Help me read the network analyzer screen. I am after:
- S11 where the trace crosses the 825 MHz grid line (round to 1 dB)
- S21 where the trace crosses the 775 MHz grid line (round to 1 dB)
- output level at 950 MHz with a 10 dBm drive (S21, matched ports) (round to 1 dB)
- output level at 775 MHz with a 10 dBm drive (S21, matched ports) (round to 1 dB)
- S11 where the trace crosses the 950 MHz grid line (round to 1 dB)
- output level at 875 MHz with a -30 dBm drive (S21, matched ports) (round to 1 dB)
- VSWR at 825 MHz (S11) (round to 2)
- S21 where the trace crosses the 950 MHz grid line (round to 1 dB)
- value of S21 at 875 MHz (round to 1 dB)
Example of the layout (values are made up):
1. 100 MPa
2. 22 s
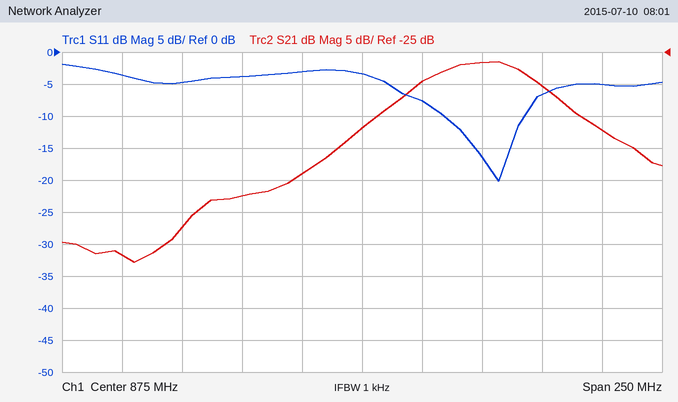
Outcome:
1. -4 dB
2. -57 dB
3. -20 dBm
4. -47 dBm
5. -7 dB
6. -67 dBm
7. 4
8. -30 dB
9. -37 dB
